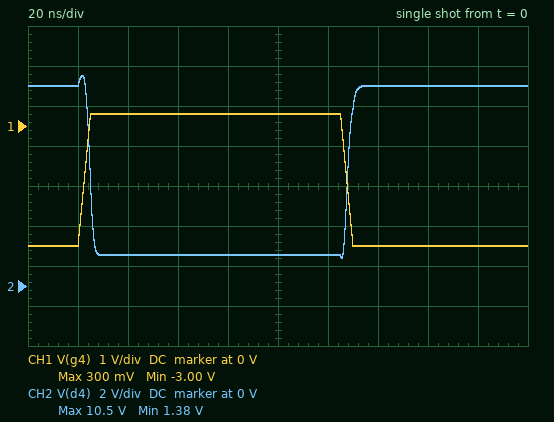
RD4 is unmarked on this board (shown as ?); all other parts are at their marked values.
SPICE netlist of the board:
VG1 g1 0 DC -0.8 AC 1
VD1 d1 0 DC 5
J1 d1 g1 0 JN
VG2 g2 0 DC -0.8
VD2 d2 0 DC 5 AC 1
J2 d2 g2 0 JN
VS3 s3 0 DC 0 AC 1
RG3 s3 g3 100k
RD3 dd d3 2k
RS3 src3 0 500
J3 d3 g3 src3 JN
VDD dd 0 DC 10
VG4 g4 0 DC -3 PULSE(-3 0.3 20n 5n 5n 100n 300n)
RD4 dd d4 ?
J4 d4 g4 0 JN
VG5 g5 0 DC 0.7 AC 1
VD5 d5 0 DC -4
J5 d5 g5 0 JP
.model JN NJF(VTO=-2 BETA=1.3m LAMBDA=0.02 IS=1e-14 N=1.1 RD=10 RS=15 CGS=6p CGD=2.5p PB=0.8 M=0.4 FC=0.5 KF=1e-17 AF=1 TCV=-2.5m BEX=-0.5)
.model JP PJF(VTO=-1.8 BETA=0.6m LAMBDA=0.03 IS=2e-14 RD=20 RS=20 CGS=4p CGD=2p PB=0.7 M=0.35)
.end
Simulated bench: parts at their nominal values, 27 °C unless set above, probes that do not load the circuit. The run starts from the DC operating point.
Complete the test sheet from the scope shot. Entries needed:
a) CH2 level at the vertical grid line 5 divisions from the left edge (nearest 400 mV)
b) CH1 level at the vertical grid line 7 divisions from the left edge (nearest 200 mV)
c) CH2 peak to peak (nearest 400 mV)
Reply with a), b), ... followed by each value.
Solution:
a) 1.6 V
b) -3.0 V
c) 9.2 V
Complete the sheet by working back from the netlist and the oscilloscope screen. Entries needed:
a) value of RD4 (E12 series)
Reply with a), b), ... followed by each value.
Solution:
a) 1.5 kΩ
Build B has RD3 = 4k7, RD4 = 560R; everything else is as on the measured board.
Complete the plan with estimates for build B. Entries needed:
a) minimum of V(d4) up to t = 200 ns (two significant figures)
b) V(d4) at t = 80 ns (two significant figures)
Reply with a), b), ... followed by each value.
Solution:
a) 6.0 V
b) 6.1 V
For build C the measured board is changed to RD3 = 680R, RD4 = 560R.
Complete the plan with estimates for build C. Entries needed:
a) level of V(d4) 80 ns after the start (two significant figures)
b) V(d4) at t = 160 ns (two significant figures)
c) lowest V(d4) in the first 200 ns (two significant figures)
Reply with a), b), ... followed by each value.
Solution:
a) 6.1 V
b) 10 V
c) 6.0 V
